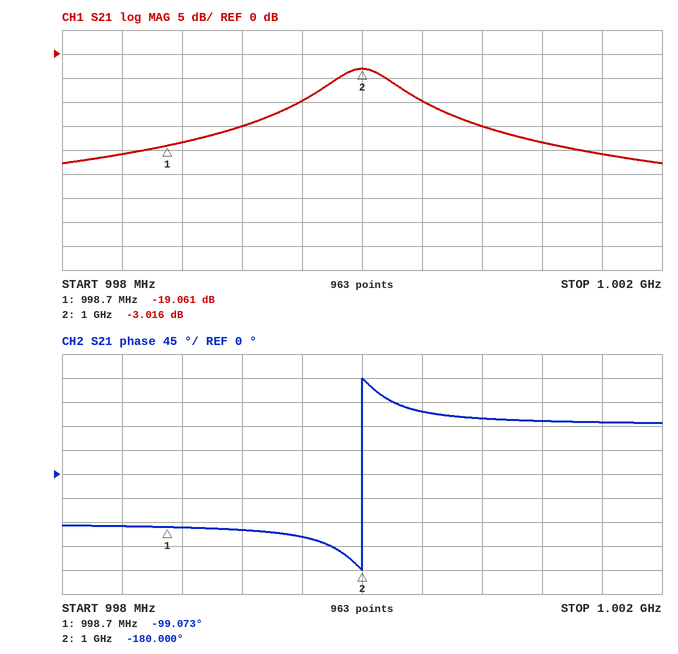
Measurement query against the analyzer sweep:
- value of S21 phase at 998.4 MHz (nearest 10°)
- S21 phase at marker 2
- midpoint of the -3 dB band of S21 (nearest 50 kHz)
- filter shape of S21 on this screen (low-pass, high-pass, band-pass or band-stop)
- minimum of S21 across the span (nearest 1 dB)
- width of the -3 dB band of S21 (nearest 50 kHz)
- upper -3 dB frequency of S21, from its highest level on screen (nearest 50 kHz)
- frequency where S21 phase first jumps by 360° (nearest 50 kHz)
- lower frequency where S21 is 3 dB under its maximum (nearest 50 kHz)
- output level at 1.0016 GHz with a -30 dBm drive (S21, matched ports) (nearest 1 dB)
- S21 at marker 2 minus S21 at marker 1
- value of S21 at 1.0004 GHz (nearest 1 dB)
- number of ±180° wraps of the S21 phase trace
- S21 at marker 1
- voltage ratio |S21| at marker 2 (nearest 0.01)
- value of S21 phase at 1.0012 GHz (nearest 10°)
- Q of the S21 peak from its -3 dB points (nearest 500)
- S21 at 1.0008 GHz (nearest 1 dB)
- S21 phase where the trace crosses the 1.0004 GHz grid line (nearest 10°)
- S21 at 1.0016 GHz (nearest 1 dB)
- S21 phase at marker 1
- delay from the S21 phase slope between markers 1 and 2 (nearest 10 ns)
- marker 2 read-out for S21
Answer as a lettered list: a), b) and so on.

a) -100°
b) -180.000°
c) 1.00000 GHz
d) band-pass
e) -23 dB
f) 400 kHz
g) 1.00020 GHz
h) 1.00000 GHz
i) 999.80 MHz
j) -51 dBm
k) 16.045 dB
l) -10 dB
m) 1
n) -19.061 dB
o) 0.71
p) 100°
q) 2500
r) -15 dB
s) 120°
t) -21 dB
u) -99.073°
v) 170 ns
w) -3.016 dB
